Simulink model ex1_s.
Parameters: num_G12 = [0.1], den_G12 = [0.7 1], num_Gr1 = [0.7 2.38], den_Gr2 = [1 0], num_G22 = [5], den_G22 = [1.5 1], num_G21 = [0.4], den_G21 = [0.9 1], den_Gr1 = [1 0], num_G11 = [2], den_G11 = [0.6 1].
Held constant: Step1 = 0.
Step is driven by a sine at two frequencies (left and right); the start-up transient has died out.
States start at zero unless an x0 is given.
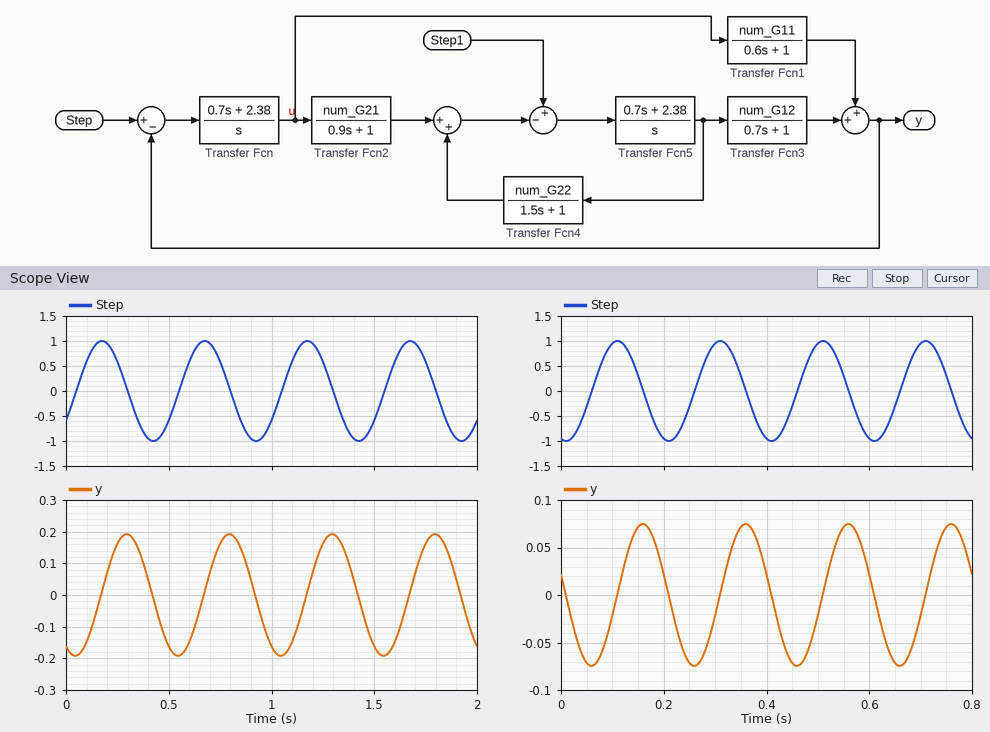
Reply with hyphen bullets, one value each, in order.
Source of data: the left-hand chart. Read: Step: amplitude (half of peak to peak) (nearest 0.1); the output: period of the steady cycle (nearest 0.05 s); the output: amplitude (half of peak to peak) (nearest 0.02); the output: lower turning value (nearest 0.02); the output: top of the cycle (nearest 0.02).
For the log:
- 1.0
- 0.50 s
- 0.20
- -0.20
- 0.20
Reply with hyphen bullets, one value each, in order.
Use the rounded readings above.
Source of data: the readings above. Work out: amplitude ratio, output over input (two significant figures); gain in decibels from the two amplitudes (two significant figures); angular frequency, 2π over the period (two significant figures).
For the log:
- 0.20
- -14 dB
- 13 rad/s
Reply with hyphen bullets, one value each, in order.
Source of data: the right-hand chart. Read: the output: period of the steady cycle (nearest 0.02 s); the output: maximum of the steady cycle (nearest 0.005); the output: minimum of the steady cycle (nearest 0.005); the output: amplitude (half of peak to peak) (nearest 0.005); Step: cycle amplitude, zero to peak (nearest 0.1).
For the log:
- 0.20 s
- 0.075
- -0.075
- 0.075
- 1.0
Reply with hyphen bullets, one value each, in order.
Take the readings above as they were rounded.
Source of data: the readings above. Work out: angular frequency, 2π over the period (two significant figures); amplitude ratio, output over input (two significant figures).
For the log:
- 31 rad/s
- 0.075
